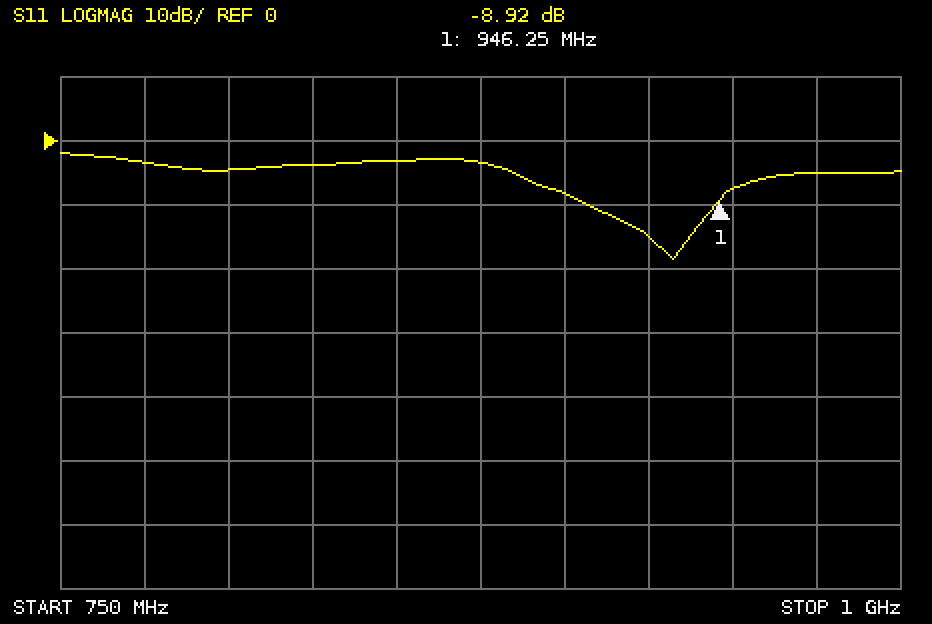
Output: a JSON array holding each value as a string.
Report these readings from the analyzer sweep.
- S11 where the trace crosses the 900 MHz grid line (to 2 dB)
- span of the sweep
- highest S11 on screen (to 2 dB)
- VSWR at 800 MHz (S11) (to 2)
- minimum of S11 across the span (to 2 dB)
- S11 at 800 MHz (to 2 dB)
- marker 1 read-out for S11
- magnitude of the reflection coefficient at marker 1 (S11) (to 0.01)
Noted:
["-8 dB", "250 MHz", "-2 dB", "4", "-18 dB", "-4 dB", "-8.92 dB", "0.36"]
